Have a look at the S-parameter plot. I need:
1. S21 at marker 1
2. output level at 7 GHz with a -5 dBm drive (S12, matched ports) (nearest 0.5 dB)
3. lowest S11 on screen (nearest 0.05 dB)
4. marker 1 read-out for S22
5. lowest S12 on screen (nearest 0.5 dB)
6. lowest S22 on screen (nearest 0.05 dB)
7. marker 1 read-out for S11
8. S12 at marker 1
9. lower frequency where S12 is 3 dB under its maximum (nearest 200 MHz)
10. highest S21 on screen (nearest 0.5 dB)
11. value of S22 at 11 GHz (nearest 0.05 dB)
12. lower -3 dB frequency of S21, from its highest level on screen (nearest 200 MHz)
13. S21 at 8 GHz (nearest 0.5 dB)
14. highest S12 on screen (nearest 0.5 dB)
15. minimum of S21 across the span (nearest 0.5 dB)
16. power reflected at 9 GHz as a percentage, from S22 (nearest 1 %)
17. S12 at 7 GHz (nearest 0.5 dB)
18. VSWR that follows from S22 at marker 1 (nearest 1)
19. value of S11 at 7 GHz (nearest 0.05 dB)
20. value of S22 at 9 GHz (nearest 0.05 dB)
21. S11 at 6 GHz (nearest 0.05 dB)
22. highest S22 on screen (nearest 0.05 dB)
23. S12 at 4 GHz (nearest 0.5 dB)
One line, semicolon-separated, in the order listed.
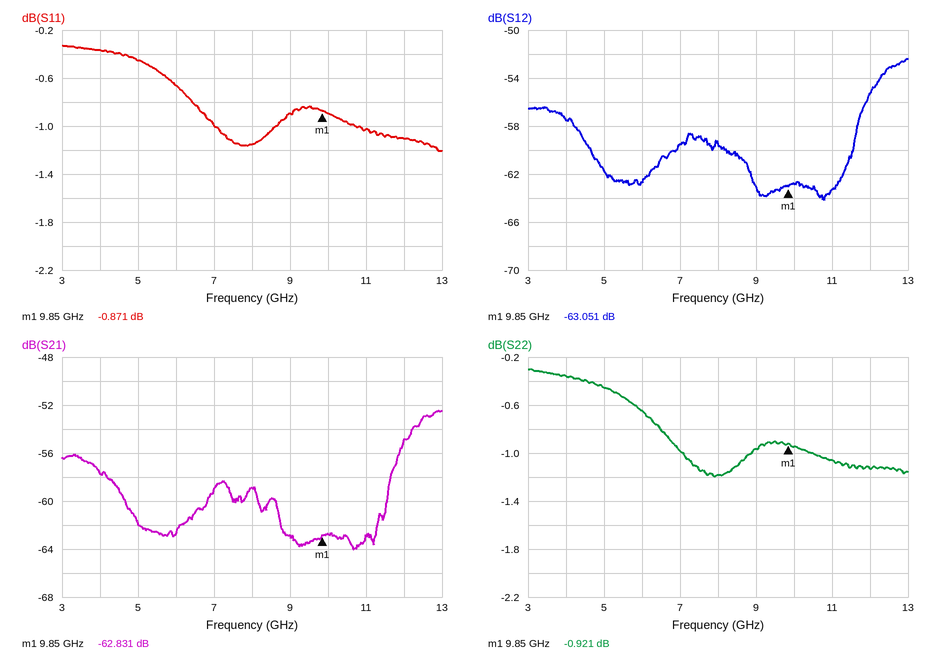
-62.831 dB; -64.5 dBm; -1.20 dB; -0.921 dB; -64.0 dB; -1.20 dB; -0.871 dB; -63.051 dB; 12.0 GHz; -52.5 dB; -1.05 dB; 12.0 GHz; -59.0 dB; -52.5 dB; -64.0 dB; 80 %; -59.5 dB; 19; -1.00 dB; -0.95 dB; -0.65 dB; -0.30 dB; -57.5 dB
